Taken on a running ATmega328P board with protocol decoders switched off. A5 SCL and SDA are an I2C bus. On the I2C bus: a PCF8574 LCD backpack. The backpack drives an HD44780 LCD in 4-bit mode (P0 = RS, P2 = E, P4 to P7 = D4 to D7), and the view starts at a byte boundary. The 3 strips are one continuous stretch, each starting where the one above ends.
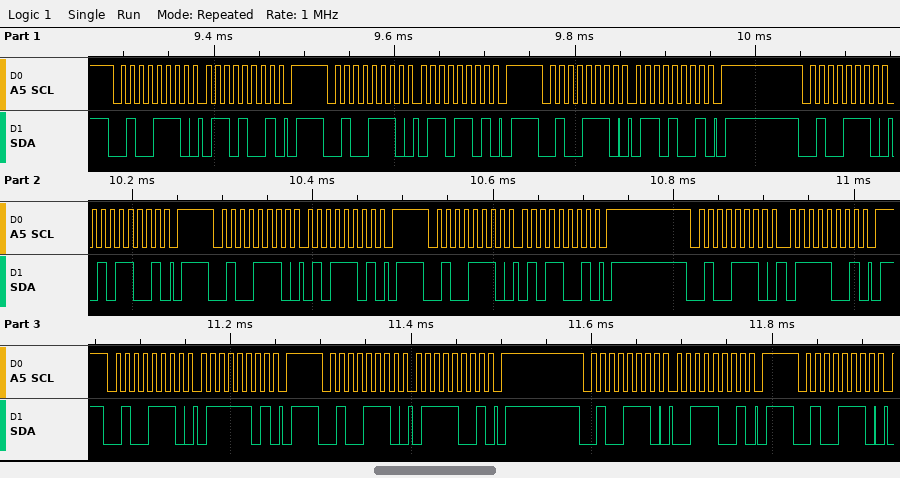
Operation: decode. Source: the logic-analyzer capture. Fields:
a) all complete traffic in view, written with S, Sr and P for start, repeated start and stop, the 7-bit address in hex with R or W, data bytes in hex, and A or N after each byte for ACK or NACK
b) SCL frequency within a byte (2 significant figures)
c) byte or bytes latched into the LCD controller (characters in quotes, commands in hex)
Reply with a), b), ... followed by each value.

a) S 27W A 69 A P S 27W A 6D A P S 27W A 69 A P S 27W A 59 A P S 27W A 5D A P S 27W A 59 A P S 27W A 79 A P S 27W A 7D A P S 27W A 79 A P S 27W A 39 A P S 27W A
b) 100 kHz
c) 'e'
